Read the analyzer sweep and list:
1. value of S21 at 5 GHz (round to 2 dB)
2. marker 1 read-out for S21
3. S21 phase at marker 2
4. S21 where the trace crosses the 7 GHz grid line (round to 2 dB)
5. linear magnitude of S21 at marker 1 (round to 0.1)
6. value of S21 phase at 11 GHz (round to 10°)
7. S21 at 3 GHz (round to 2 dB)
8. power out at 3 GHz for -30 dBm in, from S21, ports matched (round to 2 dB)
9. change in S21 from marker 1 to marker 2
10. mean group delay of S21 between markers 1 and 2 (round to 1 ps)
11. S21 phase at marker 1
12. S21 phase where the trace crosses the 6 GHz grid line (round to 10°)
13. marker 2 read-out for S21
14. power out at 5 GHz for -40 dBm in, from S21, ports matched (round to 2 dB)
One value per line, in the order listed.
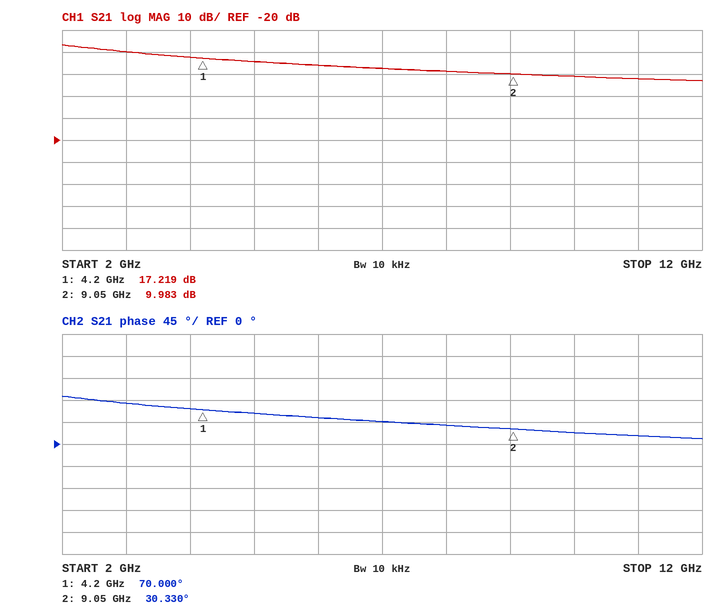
16 dB
17.219 dB
30.330°
12 dB
7.3
20°
20 dB
-10 dBm
-7.236 dB
23 ps
70.000°
50°
9.983 dB
-24 dBm
